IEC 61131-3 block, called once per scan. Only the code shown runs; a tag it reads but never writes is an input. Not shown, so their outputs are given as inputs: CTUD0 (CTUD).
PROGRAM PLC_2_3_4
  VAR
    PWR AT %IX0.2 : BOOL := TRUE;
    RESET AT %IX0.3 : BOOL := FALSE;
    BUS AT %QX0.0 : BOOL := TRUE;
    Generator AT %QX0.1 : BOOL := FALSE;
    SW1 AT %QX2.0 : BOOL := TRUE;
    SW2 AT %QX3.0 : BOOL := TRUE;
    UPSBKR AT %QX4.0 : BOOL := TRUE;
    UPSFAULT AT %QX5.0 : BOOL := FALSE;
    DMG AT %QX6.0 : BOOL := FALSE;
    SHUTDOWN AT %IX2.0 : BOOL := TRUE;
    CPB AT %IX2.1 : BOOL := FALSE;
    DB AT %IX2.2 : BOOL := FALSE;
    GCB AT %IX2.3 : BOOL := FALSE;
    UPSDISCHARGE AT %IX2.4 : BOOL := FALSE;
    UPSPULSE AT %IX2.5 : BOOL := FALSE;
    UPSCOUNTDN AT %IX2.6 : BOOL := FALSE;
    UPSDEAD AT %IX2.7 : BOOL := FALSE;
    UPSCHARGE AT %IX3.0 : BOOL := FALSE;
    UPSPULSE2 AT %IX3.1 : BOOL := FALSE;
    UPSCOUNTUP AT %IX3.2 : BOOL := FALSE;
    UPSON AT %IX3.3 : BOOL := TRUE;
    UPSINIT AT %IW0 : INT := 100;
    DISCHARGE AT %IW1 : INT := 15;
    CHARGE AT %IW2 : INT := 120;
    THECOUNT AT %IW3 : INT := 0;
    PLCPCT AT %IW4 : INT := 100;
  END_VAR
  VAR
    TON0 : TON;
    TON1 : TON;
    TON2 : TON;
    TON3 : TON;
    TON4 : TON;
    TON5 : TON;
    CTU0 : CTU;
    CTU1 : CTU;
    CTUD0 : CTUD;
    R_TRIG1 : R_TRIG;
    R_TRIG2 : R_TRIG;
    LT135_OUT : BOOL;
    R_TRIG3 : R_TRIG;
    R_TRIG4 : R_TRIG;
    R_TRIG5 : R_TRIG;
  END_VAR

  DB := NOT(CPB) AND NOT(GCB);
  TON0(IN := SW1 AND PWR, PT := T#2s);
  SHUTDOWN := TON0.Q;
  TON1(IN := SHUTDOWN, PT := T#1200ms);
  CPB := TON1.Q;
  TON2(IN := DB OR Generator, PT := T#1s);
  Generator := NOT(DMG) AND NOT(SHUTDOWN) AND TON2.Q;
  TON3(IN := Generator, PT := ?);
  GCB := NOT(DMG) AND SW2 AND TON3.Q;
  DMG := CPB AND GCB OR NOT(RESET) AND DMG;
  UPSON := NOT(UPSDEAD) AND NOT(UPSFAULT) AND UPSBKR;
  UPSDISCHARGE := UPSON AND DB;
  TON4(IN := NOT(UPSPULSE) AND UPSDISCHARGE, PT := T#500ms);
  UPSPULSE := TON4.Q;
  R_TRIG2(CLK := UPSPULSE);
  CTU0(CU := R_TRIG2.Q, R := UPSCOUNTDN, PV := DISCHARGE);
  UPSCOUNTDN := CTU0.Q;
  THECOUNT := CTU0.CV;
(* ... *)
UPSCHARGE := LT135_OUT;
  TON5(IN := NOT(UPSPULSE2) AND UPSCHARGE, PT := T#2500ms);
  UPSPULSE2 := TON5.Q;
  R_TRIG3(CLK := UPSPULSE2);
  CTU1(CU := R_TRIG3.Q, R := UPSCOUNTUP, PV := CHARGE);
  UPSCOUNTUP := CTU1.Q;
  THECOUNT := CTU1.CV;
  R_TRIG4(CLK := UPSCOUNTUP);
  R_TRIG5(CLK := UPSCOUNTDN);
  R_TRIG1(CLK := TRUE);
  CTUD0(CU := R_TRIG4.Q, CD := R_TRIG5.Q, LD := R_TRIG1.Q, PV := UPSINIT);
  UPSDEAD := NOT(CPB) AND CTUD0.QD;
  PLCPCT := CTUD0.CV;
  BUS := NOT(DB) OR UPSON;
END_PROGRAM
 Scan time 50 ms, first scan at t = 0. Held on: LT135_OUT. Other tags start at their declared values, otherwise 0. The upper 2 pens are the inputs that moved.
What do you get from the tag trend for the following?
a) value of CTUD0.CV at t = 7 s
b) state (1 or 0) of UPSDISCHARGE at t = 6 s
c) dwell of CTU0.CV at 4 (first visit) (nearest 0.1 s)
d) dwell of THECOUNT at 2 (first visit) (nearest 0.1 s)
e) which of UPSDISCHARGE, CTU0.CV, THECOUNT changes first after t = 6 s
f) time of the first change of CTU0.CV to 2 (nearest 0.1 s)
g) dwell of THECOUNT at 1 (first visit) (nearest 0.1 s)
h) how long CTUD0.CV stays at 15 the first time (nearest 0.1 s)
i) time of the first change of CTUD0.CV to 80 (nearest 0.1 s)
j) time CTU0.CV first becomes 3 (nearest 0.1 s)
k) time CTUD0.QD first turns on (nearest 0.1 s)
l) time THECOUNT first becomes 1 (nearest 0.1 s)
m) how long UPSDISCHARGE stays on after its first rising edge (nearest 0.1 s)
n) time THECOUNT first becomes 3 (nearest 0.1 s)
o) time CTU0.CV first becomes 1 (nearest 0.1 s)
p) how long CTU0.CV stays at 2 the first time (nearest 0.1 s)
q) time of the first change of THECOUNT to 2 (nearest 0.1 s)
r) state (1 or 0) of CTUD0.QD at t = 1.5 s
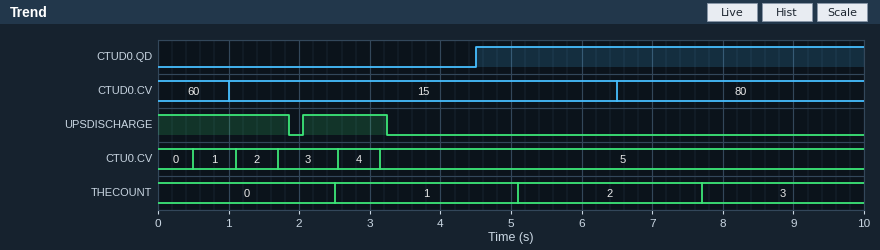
80
0
0.6 s
2.6 s
THECOUNT
1.1 s
2.6 s
5.5 s
6.5 s
1.7 s
4.5 s
2.5 s
1.2 s
7.7 s
0.5 s
0.6 s
5.1 s
0
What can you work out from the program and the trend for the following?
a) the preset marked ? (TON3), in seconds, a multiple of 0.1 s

0.8 s
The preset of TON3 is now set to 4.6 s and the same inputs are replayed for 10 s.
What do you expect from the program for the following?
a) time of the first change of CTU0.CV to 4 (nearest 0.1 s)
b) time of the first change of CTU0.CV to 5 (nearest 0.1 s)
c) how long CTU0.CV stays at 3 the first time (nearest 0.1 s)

2.3 s
2.9 s
0.6 s
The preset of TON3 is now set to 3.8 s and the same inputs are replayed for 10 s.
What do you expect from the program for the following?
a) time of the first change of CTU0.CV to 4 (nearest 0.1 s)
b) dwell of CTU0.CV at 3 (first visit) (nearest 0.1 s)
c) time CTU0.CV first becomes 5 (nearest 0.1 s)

2.3 s
0.6 s
2.9 s
